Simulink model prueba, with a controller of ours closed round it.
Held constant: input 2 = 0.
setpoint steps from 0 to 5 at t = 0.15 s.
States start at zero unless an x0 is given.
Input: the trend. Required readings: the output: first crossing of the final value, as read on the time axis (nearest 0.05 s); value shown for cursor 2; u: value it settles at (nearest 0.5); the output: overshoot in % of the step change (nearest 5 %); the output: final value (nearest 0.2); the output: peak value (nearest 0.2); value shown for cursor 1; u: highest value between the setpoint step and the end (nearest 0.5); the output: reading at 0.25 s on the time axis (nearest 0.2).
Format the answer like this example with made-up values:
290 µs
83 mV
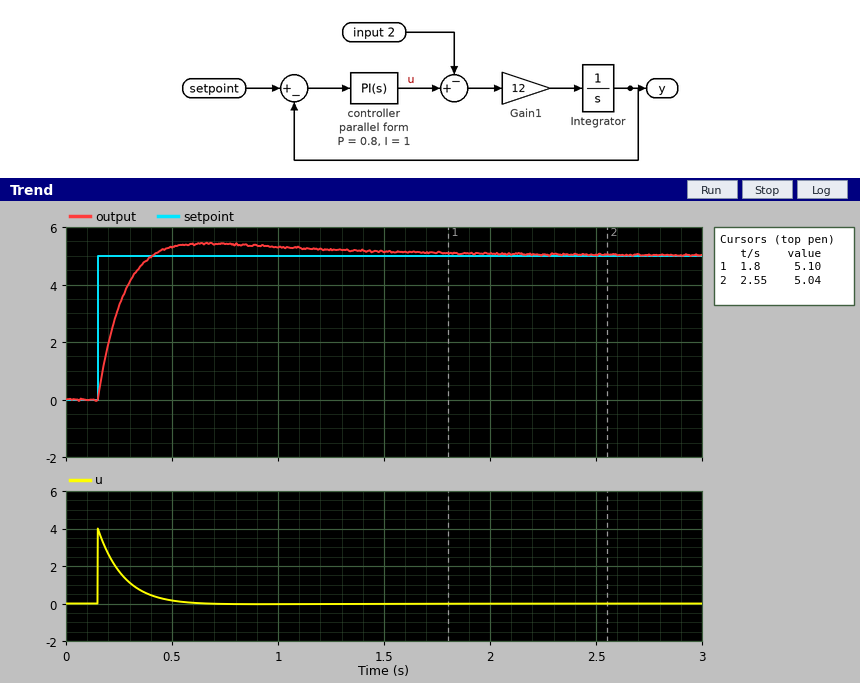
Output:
0.40 s
5.04
0.0
10 %
5.0
5.4
5.10
4.0
3.2
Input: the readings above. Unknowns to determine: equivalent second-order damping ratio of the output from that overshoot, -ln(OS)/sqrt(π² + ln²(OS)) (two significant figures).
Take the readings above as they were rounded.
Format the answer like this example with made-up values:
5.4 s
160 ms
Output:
0.59
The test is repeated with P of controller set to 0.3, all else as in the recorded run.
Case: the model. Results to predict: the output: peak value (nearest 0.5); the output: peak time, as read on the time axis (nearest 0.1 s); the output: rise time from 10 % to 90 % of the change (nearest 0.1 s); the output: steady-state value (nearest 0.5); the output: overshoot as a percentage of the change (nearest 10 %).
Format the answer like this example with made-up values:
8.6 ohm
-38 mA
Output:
6.5
0.8 s
0.3 s
5.0
30 %
